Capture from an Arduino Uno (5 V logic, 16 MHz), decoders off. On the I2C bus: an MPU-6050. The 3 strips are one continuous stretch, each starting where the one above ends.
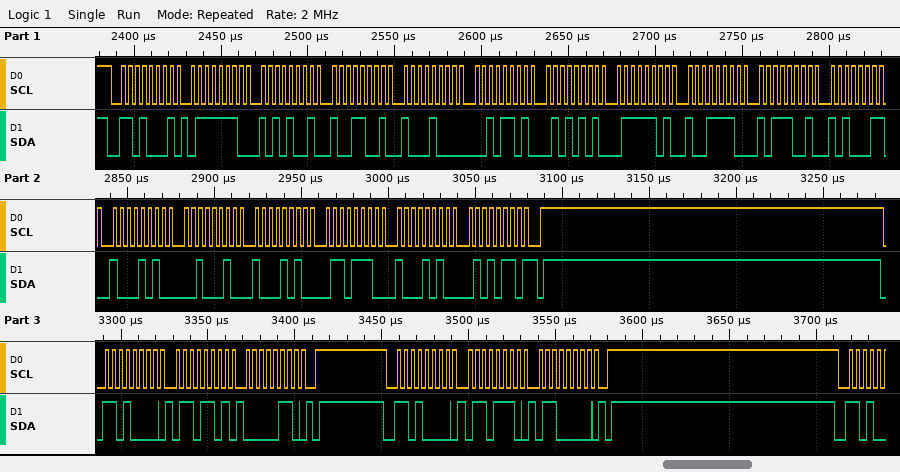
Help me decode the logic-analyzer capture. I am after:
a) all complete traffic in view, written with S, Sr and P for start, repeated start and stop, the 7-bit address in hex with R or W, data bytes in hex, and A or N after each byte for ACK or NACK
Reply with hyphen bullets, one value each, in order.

- S 68R A 7E A A9 A 99 A 88 A 2D A 55 A 7D A 9E A B9 A A3 A 8A A 22 A 8A A 6E A 8A A 56 N P S 68W A 6D A 06 A P S 68W A 6E A 60 A P
